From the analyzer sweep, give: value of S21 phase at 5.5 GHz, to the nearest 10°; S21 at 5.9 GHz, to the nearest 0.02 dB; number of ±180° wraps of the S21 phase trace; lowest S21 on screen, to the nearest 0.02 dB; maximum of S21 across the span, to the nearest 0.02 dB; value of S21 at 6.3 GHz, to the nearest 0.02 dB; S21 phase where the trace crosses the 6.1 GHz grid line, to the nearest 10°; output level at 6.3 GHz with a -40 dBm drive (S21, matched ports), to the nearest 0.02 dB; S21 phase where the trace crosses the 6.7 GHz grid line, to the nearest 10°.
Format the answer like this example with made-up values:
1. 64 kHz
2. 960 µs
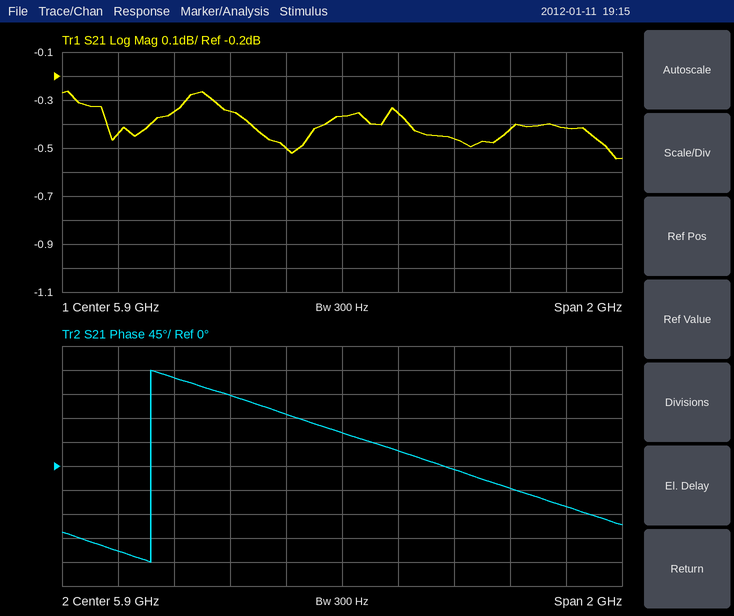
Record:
1. 130°
2. -0.36 dB
3. 1
4. -0.54 dB
5. -0.26 dB
6. -0.46 dB
7. 30°
8. -40.46 dBm
9. -80°
